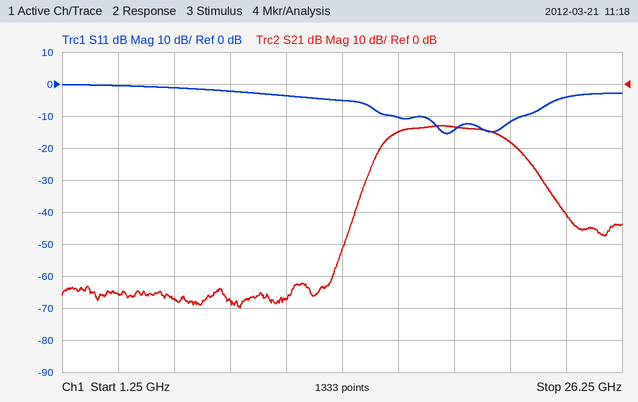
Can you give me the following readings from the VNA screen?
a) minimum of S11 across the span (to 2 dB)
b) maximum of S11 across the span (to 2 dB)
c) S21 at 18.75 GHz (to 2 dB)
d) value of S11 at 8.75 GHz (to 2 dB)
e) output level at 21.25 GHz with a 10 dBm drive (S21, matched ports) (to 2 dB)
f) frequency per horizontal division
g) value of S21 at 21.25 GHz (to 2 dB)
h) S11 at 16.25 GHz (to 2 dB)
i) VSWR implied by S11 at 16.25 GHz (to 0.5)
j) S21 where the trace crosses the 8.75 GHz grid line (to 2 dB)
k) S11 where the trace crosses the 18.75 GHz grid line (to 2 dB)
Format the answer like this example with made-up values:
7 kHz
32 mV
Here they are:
-16 dB
0 dB
-14 dB
-2 dB
-8 dBm
2.5 GHz
-18 dB
-10 dB
2.0
-68 dB
-14 dB
